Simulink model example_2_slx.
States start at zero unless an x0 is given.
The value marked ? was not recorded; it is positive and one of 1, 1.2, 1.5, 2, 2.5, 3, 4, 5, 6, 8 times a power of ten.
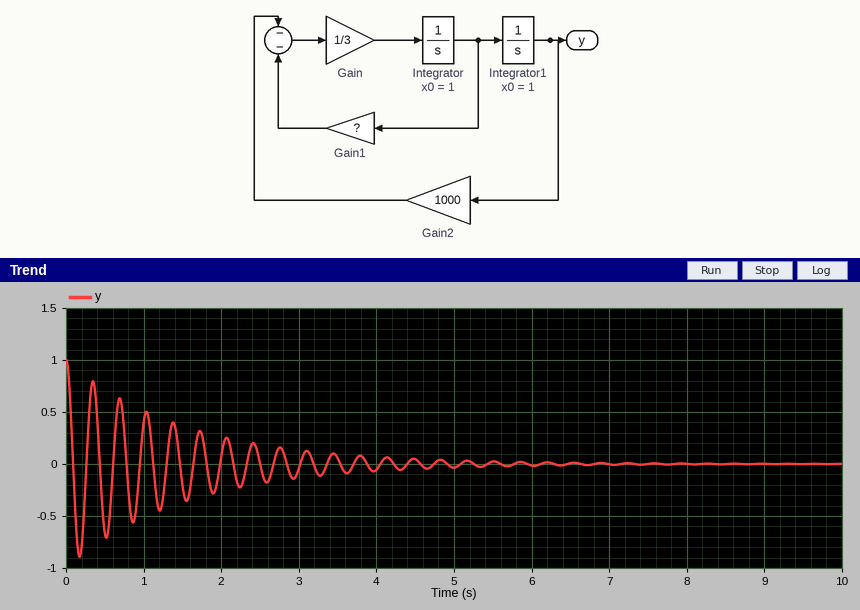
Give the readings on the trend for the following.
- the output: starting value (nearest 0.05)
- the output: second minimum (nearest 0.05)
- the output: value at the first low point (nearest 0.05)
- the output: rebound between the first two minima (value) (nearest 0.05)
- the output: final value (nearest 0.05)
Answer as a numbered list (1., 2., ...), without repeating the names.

1. 1.00
2. -0.70
3. -0.90
4. 0.80
5. 0.00
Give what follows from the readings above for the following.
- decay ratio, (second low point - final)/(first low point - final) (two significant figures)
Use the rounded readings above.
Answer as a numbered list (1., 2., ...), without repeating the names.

1. 0.78
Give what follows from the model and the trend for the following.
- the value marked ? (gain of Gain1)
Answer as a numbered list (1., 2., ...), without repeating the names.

1. 4
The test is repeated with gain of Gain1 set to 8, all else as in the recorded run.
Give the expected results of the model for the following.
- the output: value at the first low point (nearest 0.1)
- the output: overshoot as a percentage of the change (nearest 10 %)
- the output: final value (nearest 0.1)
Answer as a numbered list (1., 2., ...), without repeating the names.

1. -0.8
2. 80 %
3. 0.0
